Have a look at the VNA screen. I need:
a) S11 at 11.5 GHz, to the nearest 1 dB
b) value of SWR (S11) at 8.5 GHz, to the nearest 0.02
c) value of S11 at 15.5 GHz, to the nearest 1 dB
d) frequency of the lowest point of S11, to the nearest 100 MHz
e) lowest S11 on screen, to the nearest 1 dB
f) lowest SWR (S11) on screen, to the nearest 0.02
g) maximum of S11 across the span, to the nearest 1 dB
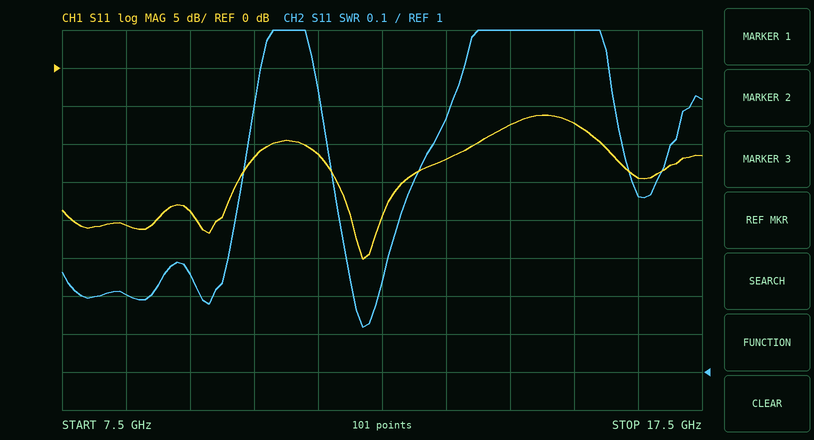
-11 dB
1.20
-7 dB
12.2 GHz
-25 dB
1.12
-6 dB
